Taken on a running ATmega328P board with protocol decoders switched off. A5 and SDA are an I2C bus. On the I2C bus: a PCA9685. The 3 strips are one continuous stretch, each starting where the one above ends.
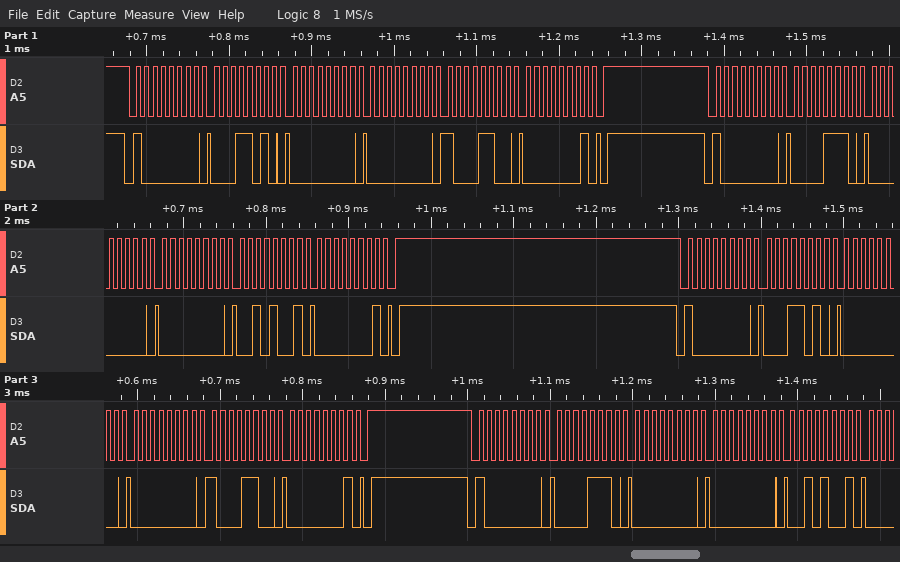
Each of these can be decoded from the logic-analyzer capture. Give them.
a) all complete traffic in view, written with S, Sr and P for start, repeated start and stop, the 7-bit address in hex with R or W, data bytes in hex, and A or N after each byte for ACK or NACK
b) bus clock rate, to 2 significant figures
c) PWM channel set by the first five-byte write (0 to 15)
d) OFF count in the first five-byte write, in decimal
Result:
S 40W A 1A A 00 A 00 A 8C A 01 A P S 40W A 0E A 00 A 00 A 29 A 01 A P S 40W A 1A A 00 A 00 A 8C A 01 A P S 40W A 0E A 00 A 00 A 29 A
100 kHz
5
396
